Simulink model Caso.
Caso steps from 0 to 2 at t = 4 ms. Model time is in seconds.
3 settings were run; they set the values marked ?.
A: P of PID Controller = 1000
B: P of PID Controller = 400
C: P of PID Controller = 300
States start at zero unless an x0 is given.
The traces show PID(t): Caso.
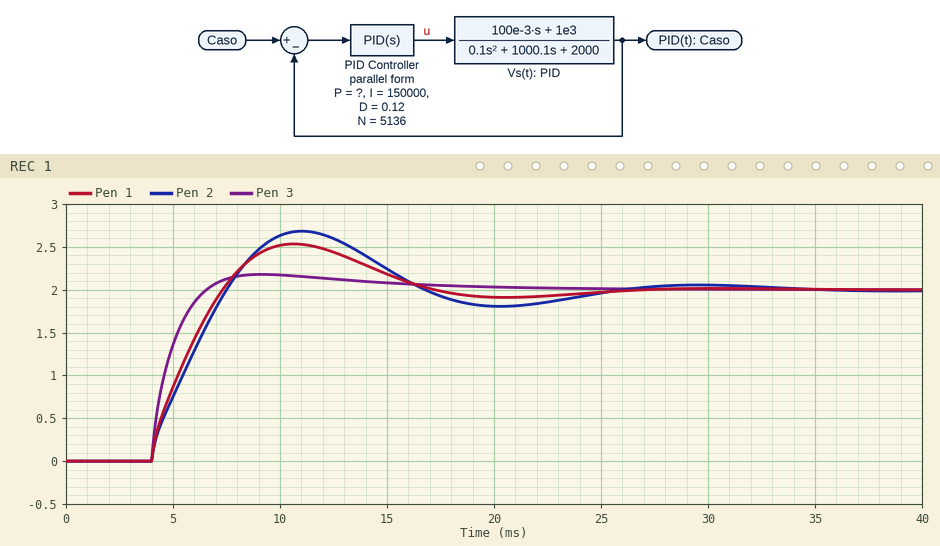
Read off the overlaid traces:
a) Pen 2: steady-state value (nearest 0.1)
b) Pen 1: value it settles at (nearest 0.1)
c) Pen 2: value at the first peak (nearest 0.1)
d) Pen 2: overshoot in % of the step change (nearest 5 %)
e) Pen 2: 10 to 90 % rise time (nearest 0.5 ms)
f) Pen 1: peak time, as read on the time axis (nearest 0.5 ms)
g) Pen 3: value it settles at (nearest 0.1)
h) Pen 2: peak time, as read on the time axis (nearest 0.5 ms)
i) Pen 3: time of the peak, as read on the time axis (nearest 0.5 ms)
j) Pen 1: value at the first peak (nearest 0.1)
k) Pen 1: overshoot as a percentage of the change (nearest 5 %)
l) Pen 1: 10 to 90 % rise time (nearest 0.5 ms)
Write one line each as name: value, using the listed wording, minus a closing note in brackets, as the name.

Pen 2: steady-state value: 2.0
Pen 1: value it settles at: 2.0
Pen 2: value at the first peak: 2.7
Pen 2: overshoot in % of the step change: 35 %
Pen 2: 10 to 90 % rise time: 3.0 ms
Pen 1: peak time, as read on the time axis: 10.5 ms
Pen 3: value it settles at: 2.0
Pen 2: peak time, as read on the time axis: 11.0 ms
Pen 3: time of the peak, as read on the time axis: 9.0 ms
Pen 1: value at the first peak: 2.5
Pen 1: overshoot as a percentage of the change: 25 %
Pen 1: 10 to 90 % rise time: 2.5 ms
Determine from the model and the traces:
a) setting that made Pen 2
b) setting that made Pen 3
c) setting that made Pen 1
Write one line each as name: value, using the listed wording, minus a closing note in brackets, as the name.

setting that made Pen 2: C
setting that made Pen 3: A
setting that made Pen 1: B
